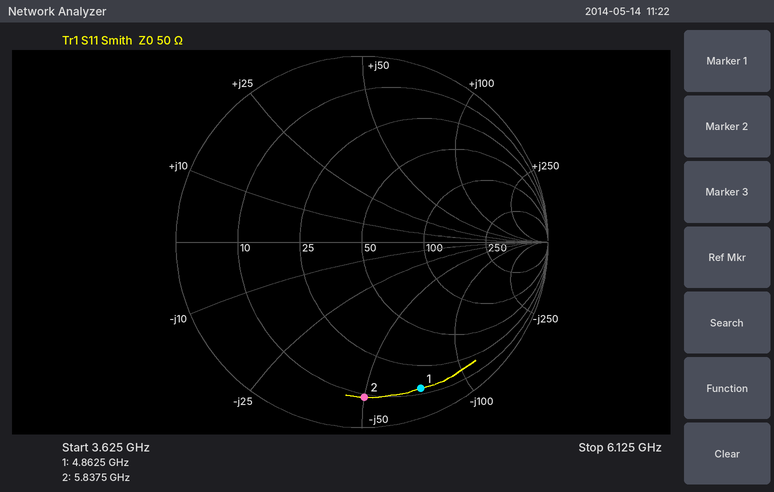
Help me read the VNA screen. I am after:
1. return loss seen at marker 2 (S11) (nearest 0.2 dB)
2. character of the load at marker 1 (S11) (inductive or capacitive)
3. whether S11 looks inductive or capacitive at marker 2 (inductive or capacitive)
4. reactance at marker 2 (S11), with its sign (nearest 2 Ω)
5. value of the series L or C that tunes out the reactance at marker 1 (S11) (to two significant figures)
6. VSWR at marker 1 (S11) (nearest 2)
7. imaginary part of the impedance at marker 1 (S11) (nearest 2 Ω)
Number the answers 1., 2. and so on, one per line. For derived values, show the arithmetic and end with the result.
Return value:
1. 1.6 dB
2. capacitive
3. capacitive
4. -50 Ω
5. L = 72 Ω/(2π × 4.8625 GHz) ≈ 2.4 nH
6. 12
7. -72 Ω
